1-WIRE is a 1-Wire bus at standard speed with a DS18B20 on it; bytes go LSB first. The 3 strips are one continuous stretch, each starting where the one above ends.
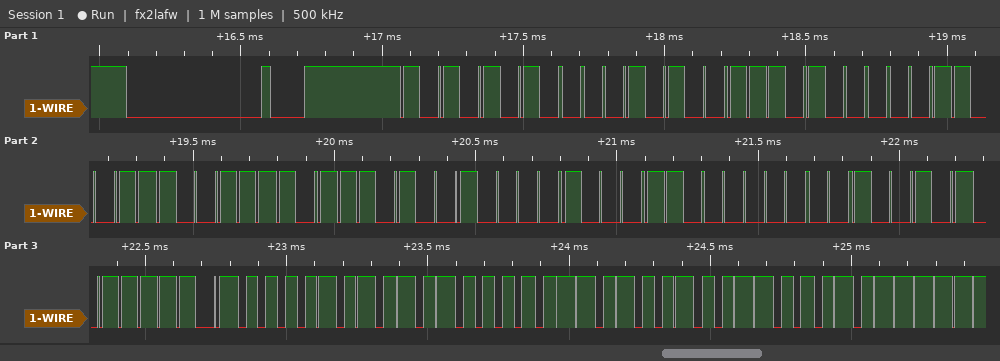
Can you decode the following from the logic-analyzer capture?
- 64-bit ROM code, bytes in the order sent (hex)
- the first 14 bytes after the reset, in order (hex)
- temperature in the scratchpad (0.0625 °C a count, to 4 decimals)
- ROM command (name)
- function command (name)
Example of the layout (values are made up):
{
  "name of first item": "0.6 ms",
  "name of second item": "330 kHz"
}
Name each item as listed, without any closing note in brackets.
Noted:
{
  "64-bit ROM code, bytes in the order sent": "28 17 CC 79 97 10 03 A4",
  "the first 14 bytes after the reset, in order": "55 28 17 CC 79 97 10 03 A4 BE 50 05 4B 46",
  "temperature in the scratchpad": "85.0000 °C",
  "ROM command": "Match ROM",
  "function command": "Read Scratchpad"
}
